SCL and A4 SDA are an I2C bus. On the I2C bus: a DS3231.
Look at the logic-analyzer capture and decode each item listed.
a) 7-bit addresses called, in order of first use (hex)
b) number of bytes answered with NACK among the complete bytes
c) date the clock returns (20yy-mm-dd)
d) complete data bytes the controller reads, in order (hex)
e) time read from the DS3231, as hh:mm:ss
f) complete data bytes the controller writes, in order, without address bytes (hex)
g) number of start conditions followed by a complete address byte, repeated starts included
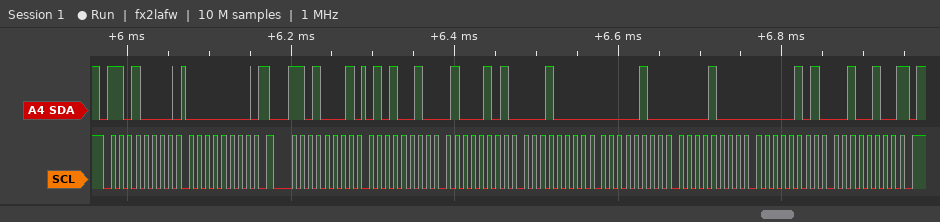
0x68
1
2024-05-08
52 45 10 04 08 05 24
10:45:52
00
2
